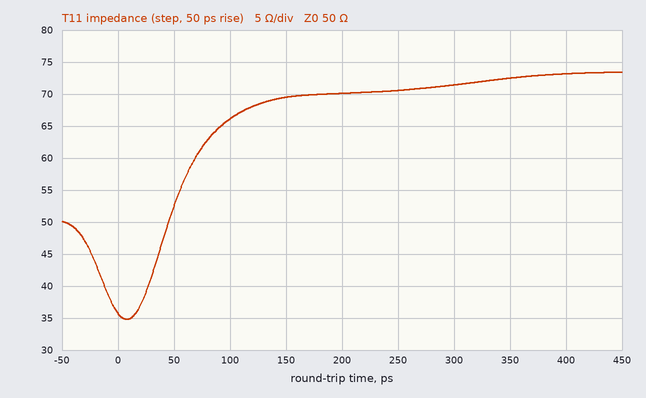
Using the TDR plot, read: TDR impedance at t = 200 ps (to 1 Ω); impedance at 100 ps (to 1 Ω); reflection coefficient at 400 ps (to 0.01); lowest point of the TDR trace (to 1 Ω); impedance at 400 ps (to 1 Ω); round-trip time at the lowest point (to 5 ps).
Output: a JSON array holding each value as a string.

["70 Ω", "66 Ω", "+0.19", "35 Ω", "73 Ω", "10 ps"]
